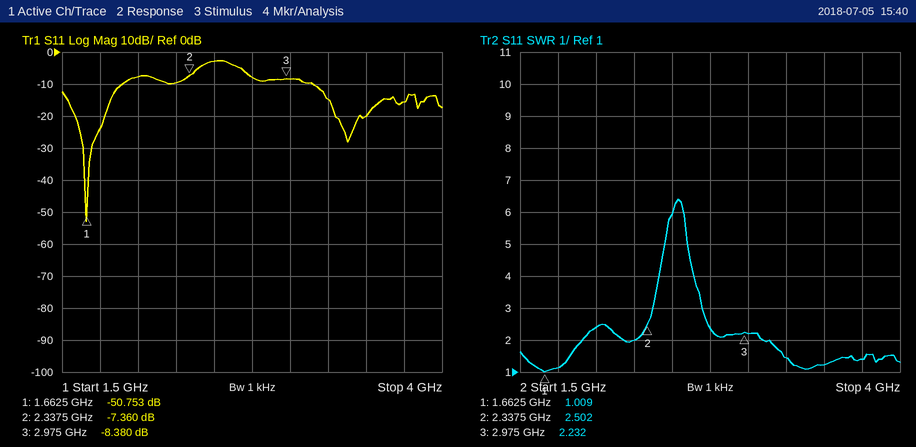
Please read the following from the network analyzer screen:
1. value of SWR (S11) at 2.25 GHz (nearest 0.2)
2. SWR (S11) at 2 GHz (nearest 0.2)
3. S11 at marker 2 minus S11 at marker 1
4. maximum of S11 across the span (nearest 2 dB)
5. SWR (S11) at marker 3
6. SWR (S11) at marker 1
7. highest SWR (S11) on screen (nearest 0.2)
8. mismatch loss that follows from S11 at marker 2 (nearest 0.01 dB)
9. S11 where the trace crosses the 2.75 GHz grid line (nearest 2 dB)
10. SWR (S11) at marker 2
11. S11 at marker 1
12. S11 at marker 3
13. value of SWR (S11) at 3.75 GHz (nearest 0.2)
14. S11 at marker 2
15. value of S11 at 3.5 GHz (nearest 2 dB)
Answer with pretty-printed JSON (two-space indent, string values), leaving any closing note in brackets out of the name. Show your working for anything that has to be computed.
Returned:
{
  "value of SWR (S11) at 2.25 GHz": "2.0",
  "SWR (S11) at 2 GHz": "2.4",
  "S11 at marker 2 minus S11 at marker 1": "-7.36 − (-50.753) = 43.393 dB",
  "maximum of S11 across the span": "-2 dB",
  "SWR (S11) at marker 3": "2.232",
  "SWR (S11) at marker 1": "1.009",
  "highest SWR (S11) on screen": "6.4",
  "mismatch loss that follows from S11 at marker 2": "−10 log10(1 − 10^(-7.36/10)) ≈ 0.88 dB",
  "S11 where the trace crosses the 2.75 GHz grid line": "-8 dB",
  "SWR (S11) at marker 2": "2.502",
  "S11 at marker 1": "-50.753 dB",
  "S11 at marker 3": "-8.380 dB",
  "value of SWR (S11) at 3.75 GHz": "1.4",
  "S11 at marker 2": "-7.360 dB",
  "value of S11 at 3.5 GHz": "-20 dB"
}
